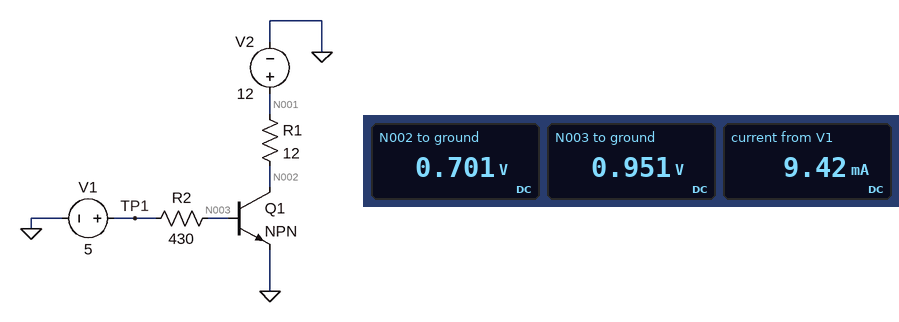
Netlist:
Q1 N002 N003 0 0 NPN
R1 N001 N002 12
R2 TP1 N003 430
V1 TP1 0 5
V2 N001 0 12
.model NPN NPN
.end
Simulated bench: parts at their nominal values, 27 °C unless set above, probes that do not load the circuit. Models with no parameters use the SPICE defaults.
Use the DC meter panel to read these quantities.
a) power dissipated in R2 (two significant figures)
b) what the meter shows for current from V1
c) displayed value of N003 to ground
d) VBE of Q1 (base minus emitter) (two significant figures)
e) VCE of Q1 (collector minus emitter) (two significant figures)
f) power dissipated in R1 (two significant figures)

38 mW
9.42 mA
0.951 V
950 mV
700 mV
11 W
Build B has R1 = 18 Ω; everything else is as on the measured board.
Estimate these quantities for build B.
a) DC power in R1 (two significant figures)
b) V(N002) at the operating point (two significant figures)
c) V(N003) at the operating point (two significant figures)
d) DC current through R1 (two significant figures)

7.8 W
140 mV
940 mV
660 mA
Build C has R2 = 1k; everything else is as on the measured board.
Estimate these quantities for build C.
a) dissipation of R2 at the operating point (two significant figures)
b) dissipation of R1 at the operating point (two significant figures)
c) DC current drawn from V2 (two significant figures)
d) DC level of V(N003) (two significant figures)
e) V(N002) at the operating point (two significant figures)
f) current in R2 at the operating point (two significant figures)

17 mW
2.0 W
410 mA
930 mV
7.1 V
4.1 mA
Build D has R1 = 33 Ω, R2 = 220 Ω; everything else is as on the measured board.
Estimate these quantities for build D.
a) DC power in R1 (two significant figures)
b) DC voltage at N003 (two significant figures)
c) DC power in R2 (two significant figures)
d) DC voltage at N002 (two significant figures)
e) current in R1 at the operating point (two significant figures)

4.3 W
930 mV
75 mW
85 mV
360 mA
